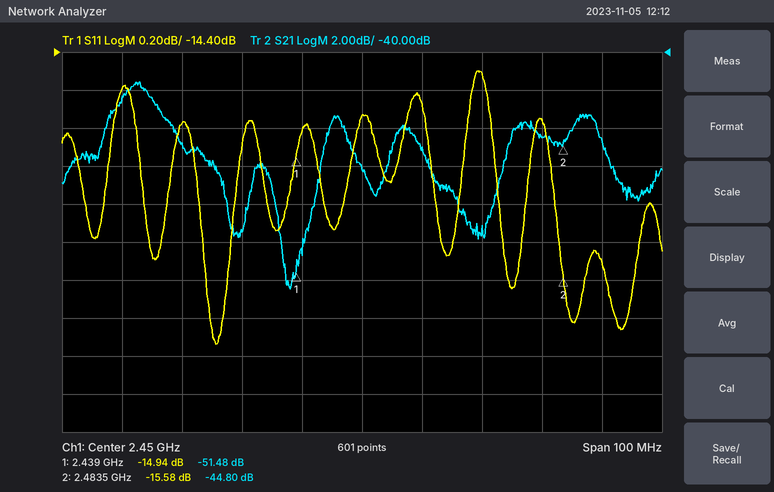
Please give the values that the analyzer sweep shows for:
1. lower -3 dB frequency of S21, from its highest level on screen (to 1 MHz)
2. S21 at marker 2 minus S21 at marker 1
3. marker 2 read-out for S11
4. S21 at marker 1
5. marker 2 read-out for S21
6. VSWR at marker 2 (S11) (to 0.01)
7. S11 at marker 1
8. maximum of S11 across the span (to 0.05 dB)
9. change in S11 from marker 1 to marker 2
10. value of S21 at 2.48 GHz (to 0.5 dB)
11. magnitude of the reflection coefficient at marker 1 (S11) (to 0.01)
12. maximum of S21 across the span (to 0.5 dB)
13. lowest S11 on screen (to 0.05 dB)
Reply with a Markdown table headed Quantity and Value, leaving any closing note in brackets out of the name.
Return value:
| Quantity | Value |
|---|---|
| lower -3 dB frequency of S21, from its highest level on screen | 2.407 GHz |
| S21 at marker 2 minus S21 at marker 1 | 6.68 dB |
| marker 2 read-out for S11 | -15.58 dB |
| S21 at marker 1 | -51.48 dB |
| marker 2 read-out for S21 | -44.80 dB |
| VSWR at marker 2 (S11) | 1.40 |
| S11 at marker 1 | -14.94 dB |
| maximum of S11 across the span | -14.50 dB |
| change in S11 from marker 1 to marker 2 | -0.64 dB |
| value of S21 at 2.48 GHz | -44.5 dB |
| magnitude of the reflection coefficient at marker 1 (S11) | 0.18 |
| maximum of S21 across the span | -41.5 dB |
| lowest S11 on screen | -15.95 dB |
